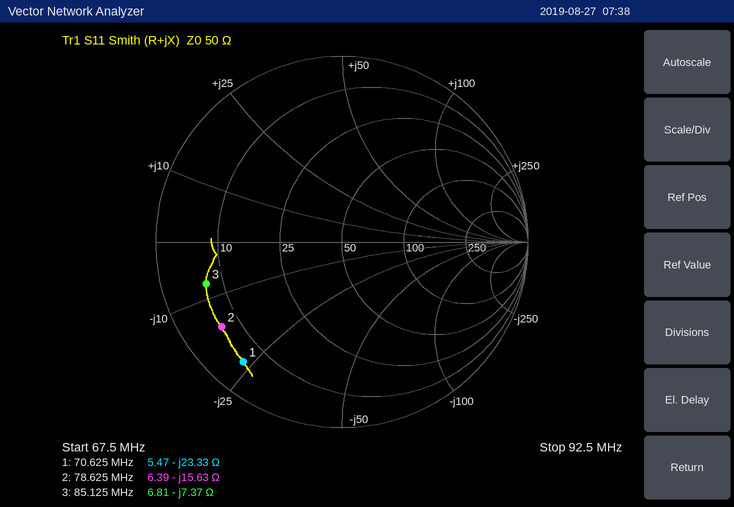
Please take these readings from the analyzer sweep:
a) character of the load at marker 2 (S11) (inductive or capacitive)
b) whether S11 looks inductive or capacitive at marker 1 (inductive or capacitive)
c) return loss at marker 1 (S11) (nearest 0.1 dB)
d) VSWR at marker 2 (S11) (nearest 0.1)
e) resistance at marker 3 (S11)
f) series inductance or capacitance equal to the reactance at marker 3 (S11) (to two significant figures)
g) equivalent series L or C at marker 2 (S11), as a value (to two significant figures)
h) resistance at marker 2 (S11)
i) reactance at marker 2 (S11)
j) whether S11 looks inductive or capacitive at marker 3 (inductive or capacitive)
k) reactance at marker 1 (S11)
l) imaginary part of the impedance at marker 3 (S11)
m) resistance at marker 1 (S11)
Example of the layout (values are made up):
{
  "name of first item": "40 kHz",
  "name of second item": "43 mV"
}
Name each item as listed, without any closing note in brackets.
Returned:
{
  "character of the load at marker 2 (S11)": "capacitive",
  "whether S11 looks inductive or capacitive at marker 1": "capacitive",
  "return loss at marker 1 (S11)": "1.6 dB",
  "VSWR at marker 2 (S11)": "8.6",
  "resistance at marker 3": "6.81 Ω",
  "series inductance or capacitance equal to the reactance at marker 3 (S11)": "250 pF",
  "equivalent series L or C at marker 2 (S11), as a value": "130 pF",
  "resistance at marker 2": "6.39 Ω",
  "reactance at marker 2": "-15.63 Ω",
  "whether S11 looks inductive or capacitive at marker 3": "capacitive",
  "reactance at marker 1": "-23.33 Ω",
  "imaginary part of the impedance at marker 3": "-7.37 Ω",
  "resistance at marker 1": "5.47 Ω"
}
